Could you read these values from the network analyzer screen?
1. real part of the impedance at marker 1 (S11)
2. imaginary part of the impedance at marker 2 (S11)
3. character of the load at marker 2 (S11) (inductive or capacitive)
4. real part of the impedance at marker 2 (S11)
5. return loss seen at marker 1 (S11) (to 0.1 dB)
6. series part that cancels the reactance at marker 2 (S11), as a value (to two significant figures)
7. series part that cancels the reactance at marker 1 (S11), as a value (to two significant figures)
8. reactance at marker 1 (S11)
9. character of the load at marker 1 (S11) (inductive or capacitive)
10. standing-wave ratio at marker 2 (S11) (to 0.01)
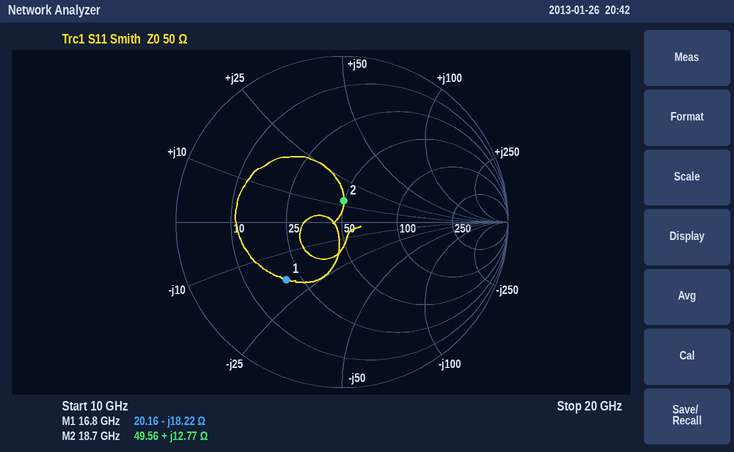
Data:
20.16 Ω
+12.77 Ω
inductive
49.56 Ω
6.3 dB
670 fF
170 pH
-18.22 Ω
capacitive
1.29
